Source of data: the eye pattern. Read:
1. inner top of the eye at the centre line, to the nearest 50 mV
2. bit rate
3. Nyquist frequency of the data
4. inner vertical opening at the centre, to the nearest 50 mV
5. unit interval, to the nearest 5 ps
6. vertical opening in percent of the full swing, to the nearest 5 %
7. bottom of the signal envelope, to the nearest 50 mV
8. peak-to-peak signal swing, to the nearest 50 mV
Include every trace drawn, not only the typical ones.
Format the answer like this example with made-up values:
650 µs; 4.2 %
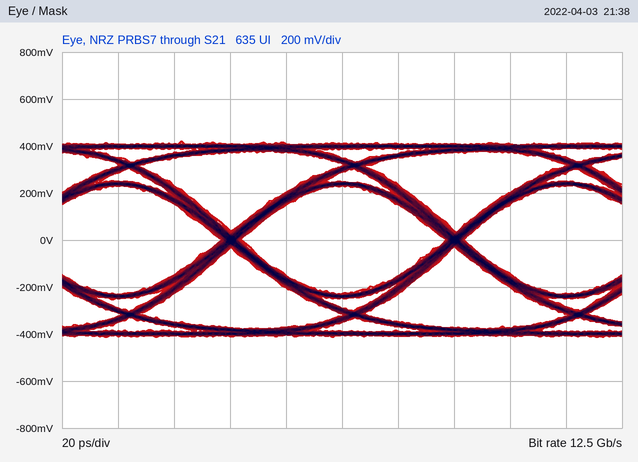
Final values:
250 mV; 12.5 Gb/s; 6.25 GHz; 450 mV; 80 ps; 55 %; -400 mV; 850 mV
